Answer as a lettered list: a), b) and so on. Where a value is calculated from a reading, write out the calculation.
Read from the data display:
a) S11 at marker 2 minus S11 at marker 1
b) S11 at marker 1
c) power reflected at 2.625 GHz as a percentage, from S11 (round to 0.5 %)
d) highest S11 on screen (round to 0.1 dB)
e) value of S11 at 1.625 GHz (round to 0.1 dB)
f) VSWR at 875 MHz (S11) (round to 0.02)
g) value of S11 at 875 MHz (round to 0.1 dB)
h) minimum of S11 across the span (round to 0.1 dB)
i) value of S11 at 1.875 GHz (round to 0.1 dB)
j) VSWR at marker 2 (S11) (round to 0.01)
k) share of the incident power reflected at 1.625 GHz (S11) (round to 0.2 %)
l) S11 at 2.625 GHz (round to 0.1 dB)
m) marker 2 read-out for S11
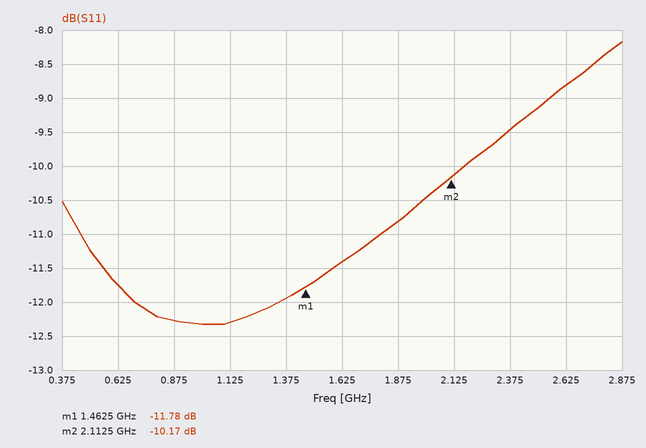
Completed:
a) -10.17 − (-11.78) = 1.61 dB
b) -11.78 dB
c) 10^(-8.8/10) ≈ 13.2 %, so 13.0 % to the nearest 0.5 %
d) -8.2 dB
e) -11.4 dB
f) |Γ| = 10^(-12.3/20) = 0.2427; VSWR = (1 + 0.2427)/(1 − 0.2427) ≈ 1.64
g) -12.3 dB
h) -12.3 dB
i) -10.8 dB
j) (1 + 0.3101)/(1 − 0.3101) ≈ 1.90
k) 10^(-11.4/10) ≈ 7.2 %
l) -8.8 dB
m) -10.17 dB
